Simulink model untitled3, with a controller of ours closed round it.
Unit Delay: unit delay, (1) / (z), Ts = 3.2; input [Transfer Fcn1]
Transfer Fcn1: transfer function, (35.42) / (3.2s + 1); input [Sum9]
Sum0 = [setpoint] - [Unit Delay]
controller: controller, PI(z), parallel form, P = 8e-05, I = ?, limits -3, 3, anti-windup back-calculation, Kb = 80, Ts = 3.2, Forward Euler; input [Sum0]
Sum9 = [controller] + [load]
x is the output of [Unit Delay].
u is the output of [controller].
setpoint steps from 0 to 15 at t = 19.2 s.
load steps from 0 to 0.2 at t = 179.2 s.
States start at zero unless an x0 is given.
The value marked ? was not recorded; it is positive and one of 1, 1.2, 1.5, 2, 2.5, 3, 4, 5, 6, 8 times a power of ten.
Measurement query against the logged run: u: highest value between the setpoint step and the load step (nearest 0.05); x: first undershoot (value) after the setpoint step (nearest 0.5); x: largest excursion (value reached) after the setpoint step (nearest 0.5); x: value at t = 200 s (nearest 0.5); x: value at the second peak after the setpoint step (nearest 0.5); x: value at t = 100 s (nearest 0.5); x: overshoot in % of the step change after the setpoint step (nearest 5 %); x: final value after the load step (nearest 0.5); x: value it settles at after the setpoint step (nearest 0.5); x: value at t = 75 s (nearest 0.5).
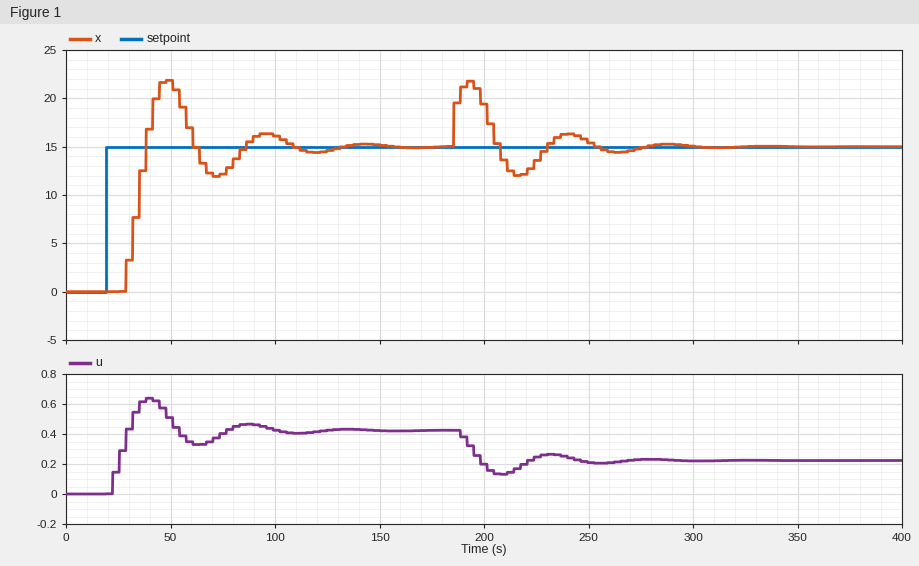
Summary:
0.65
12.0
22.0
19.5
16.5
16.0
45 %
15.0
15.0
12.0
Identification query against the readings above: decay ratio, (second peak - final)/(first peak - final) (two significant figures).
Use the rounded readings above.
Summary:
0.21
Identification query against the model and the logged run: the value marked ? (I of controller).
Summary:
0.003
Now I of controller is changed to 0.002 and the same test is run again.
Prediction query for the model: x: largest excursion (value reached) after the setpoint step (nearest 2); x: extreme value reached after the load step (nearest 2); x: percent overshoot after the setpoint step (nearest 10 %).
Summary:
18
22
20 %
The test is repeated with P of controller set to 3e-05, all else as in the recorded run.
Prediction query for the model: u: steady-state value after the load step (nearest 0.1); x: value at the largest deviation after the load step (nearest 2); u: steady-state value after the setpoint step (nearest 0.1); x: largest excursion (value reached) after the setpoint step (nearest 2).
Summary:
0.2
22
0.4
22
